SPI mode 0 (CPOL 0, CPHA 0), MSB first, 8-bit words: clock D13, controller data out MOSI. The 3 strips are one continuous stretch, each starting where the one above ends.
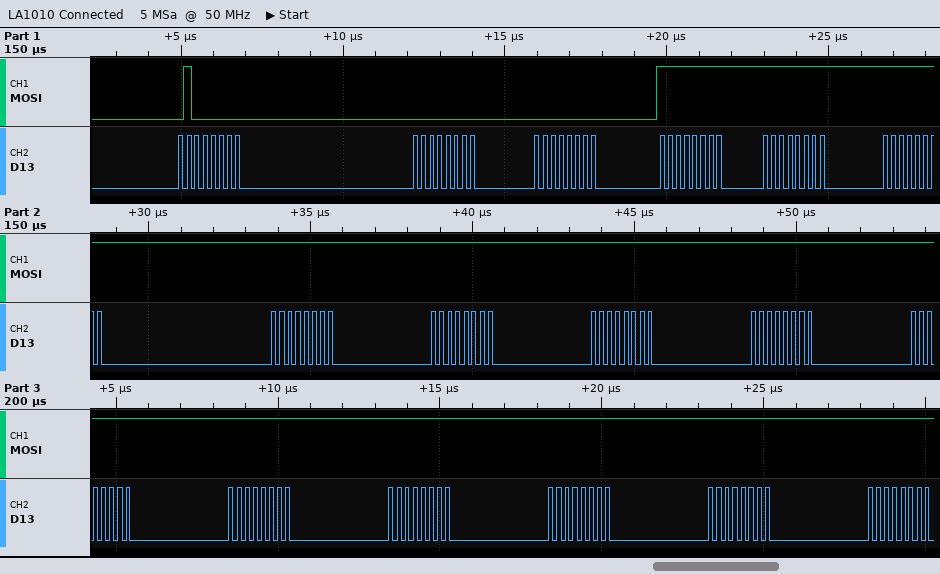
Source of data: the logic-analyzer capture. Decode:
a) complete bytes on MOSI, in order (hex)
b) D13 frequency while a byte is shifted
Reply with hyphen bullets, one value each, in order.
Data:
- 40 00 00 FF FF FF FF FF FF FF FF FF FF FF FF FF
- 4 MHz
